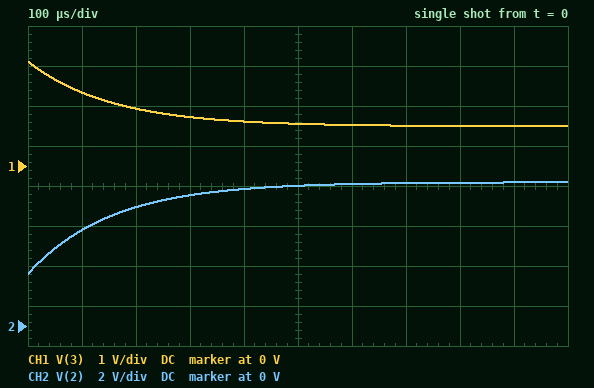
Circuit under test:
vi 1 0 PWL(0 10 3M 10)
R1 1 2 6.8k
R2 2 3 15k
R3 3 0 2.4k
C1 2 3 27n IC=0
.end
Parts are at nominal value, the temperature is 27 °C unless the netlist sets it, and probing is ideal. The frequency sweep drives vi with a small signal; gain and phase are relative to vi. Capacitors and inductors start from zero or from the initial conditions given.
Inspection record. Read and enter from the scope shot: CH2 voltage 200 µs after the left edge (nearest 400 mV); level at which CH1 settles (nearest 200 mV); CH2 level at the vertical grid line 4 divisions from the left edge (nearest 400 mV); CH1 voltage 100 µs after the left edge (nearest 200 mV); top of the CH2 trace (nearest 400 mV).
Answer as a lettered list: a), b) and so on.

a) 6.0 V
b) 1.0 V
c) 6.8 V
d) 1.8 V
e) 7.2 V
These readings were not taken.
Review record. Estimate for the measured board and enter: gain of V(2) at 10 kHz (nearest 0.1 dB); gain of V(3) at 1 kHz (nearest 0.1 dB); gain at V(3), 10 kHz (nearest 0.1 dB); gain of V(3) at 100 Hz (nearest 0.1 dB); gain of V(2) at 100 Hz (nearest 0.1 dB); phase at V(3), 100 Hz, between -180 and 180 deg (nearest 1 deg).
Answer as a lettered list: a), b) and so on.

a) -11.4 dB
b) -14.2 dB
c) -11.7 dB
d) -19.8 dB
e) -2.9 dB
f) 9 deg
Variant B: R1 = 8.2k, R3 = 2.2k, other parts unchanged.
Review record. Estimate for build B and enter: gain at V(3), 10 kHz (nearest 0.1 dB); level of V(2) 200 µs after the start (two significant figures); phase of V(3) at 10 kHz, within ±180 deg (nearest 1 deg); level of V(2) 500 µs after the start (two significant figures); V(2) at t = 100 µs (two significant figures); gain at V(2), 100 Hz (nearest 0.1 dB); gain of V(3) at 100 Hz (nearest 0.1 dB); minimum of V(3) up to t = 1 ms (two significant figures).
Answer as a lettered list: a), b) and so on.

a) -13.5 dB
b) 5.4 V
c) 3 deg
d) 6.5 V
e) 4.2 V
f) -3.4 dB
g) -21.0 dB
h) 870 mV
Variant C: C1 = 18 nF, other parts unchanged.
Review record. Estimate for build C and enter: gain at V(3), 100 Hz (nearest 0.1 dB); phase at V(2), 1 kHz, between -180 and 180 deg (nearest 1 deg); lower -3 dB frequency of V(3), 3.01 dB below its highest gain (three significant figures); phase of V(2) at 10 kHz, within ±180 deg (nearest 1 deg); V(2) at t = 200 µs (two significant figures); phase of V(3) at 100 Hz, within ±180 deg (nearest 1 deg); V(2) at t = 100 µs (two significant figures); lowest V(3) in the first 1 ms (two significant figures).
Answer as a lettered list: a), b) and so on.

a) -20.0 dB
b) -20 deg
c) 1.31 kHz
d) -14 deg
e) 6.5 V
f) 6 deg
g) 5.5 V
h) 990 mV
